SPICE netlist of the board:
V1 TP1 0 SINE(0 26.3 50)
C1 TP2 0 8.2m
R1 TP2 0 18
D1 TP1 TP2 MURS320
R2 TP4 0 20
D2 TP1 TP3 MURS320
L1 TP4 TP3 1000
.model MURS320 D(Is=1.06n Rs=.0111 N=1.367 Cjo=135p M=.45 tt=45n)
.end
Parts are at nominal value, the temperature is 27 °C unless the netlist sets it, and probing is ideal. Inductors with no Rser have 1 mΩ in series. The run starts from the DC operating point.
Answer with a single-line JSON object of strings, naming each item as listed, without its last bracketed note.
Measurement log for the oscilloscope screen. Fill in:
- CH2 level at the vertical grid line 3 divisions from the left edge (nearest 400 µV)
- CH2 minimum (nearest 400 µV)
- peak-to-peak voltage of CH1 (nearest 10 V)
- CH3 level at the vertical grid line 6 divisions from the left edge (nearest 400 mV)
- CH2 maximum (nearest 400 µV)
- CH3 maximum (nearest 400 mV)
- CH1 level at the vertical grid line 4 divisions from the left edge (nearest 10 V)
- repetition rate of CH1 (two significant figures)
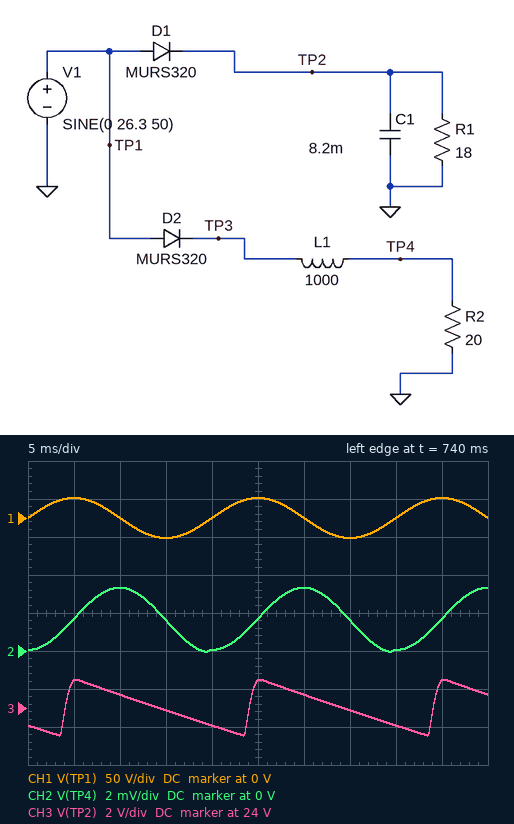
{"CH2 level at the vertical grid line 3 divisions from the left edge": "1.6 mV", "CH2 minimum": "0 V", "peak-to-peak voltage of CH1": "50 V", "CH3 level at the vertical grid line 6 divisions from the left edge": "24.8 V", "CH2 maximum": "3.2 mV", "CH3 maximum": "25.6 V", "CH1 level at the vertical grid line 4 divisions from the left edge": "0 V", "repetition rate of CH1": "50 Hz"}
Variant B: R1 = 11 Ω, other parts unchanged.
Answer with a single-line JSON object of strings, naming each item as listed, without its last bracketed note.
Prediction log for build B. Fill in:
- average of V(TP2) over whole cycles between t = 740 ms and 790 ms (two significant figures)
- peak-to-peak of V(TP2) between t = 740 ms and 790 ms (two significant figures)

{"average of V(TP2) over whole cycles between t = 740 ms and 790 ms": "23 V", "peak-to-peak of V(TP2) between t = 740 ms and 790 ms": "4.6 V"}
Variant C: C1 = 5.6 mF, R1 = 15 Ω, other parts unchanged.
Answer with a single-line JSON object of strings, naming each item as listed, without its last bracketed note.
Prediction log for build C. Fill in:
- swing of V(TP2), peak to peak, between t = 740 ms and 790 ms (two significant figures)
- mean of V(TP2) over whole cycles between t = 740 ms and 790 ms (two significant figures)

{"swing of V(TP2), peak to peak, between t = 740 ms and 790 ms": "4.9 V", "mean of V(TP2) over whole cycles between t = 740 ms and 790 ms": "23 V"}
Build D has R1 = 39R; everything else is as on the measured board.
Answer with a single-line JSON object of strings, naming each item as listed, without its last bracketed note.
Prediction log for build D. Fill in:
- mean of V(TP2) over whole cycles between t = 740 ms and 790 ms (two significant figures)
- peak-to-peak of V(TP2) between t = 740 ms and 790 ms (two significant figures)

{"mean of V(TP2) over whole cycles between t = 740 ms and 790 ms": "25 V", "peak-to-peak of V(TP2) between t = 740 ms and 790 ms": "1.4 V"}
